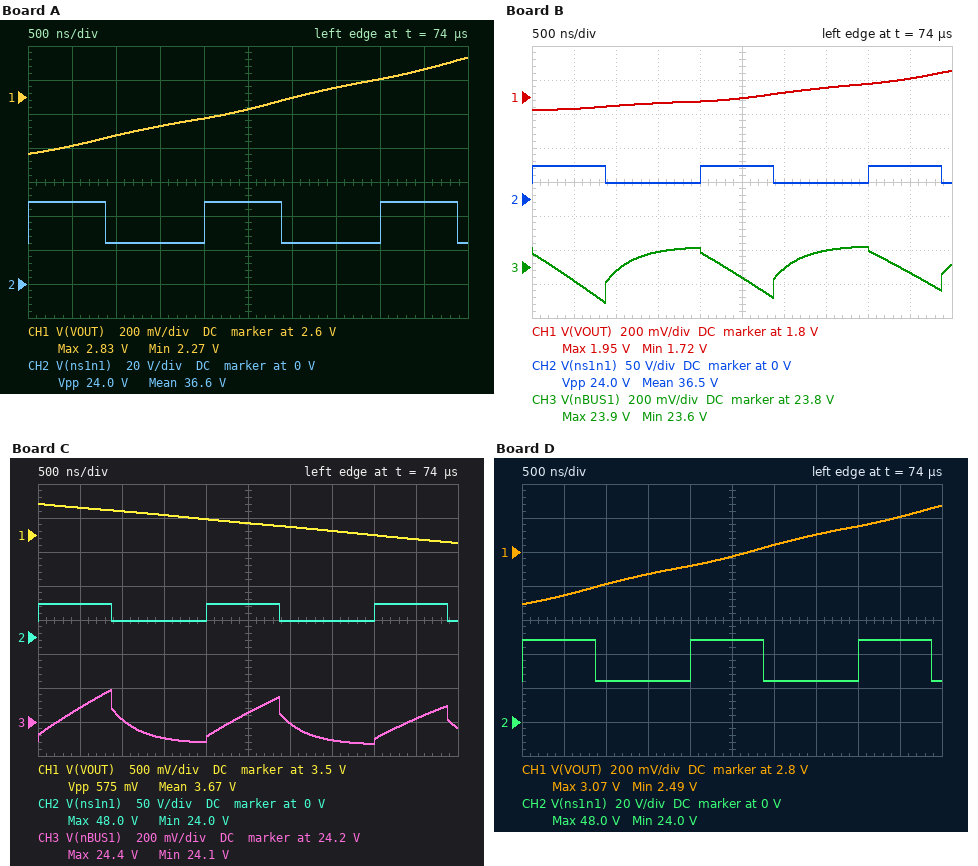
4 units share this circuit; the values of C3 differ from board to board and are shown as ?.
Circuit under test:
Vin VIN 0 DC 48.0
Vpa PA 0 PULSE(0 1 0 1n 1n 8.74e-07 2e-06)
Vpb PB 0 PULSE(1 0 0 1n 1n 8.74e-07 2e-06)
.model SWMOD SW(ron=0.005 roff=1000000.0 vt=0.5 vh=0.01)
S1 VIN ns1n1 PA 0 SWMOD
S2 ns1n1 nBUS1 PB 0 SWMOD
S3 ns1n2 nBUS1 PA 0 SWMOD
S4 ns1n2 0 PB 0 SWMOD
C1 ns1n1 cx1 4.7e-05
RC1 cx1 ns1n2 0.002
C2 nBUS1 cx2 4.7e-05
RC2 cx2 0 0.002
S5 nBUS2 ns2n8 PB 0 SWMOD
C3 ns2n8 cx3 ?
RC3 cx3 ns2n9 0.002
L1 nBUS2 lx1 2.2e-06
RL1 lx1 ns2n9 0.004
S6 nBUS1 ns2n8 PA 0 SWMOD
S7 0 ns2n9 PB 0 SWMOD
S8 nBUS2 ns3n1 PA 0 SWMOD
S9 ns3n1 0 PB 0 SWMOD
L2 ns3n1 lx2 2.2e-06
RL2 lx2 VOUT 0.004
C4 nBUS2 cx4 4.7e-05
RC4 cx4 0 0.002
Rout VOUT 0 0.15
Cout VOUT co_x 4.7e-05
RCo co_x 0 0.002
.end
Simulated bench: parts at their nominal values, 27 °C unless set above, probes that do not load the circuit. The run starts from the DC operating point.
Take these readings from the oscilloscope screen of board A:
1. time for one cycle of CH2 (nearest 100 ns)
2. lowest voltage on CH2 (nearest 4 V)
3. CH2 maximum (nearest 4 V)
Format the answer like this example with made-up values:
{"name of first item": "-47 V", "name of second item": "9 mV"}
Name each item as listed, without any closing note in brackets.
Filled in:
{"time for one cycle of CH2": "2.0 µs", "lowest voltage on CH2": "24 V", "CH2 maximum": "48 V"}
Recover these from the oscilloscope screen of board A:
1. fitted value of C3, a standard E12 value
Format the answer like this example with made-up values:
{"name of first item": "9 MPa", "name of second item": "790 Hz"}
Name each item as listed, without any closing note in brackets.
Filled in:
{"fitted value of C3, a standard E12 value": "22 µF"}
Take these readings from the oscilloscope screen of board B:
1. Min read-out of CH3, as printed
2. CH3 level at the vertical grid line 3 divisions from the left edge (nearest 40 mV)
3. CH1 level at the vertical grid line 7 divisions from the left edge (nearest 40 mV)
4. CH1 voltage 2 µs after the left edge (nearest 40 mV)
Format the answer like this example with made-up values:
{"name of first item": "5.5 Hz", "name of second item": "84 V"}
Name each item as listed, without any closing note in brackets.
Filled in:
{"Min read-out of CH3, as printed": "23.6 V", "CH3 level at the vertical grid line 3 divisions from the left edge": "23.88 V", "CH1 level at the vertical grid line 7 divisions from the left edge": "1.84 V", "CH1 voltage 2 µs after the left edge": "1.76 V"}
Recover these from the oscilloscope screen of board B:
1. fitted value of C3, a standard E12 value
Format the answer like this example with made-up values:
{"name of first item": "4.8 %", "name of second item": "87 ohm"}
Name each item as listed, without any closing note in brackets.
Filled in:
{"fitted value of C3, a standard E12 value": "39 µF"}
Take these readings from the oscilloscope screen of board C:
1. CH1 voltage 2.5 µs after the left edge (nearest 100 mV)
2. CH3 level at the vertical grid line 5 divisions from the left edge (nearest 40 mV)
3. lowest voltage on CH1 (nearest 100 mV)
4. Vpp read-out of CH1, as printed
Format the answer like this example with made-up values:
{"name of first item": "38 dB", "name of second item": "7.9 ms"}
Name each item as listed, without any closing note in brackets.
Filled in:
{"CH1 voltage 2.5 µs after the left edge": "3.7 V", "CH3 level at the vertical grid line 5 divisions from the left edge": "24.24 V", "lowest voltage on CH1": "3.4 V", "Vpp read-out of CH1, as printed": "575 mV"}
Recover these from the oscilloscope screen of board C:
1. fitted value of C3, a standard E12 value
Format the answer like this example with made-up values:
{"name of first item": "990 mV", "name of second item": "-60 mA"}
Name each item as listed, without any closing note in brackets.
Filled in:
{"fitted value of C3, a standard E12 value": "150 µF"}
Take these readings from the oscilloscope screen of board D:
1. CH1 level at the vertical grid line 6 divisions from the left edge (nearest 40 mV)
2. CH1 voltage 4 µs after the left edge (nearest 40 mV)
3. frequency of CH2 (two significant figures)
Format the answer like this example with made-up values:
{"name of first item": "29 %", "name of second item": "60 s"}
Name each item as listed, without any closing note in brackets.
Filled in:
{"CH1 level at the vertical grid line 6 divisions from the left edge": "2.84 V", "CH1 voltage 4 µs after the left edge": "2.96 V", "frequency of CH2": "500 kHz"}
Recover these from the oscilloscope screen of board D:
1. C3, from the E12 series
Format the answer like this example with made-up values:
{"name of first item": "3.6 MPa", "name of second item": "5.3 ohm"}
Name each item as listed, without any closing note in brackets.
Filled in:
{"C3, from the E12 series": "18 µF"}
